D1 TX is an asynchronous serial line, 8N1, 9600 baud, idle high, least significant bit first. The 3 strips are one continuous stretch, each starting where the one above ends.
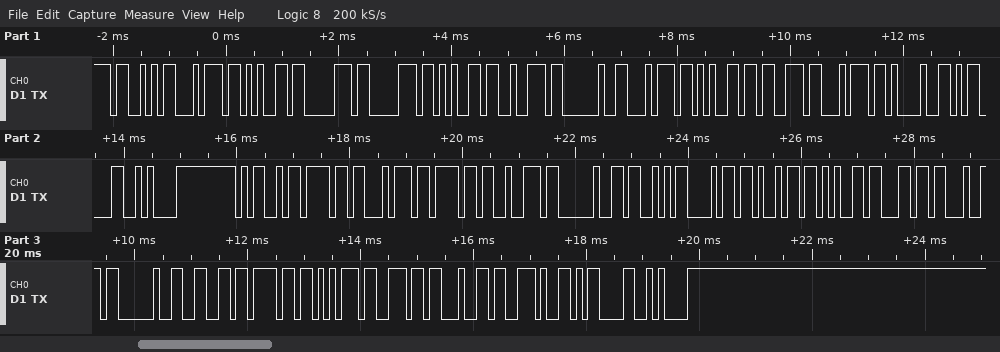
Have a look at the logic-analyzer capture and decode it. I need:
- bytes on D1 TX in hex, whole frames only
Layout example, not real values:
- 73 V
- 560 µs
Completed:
- 0x53 0x74 0x65 0x70 0x70 0x65 0x72 0x20 0x74 0x65 0x73 0x74 0x21 0x0D 0x0A 0x4D 0x6F 0x74 0x6F 0x72 0x20 0x53 0x68 0x69 0x65 0x6C 0x64 0x20 0x66 0x6F 0x75 0x6E 0x64 0x2E 0x0D 0x0A
